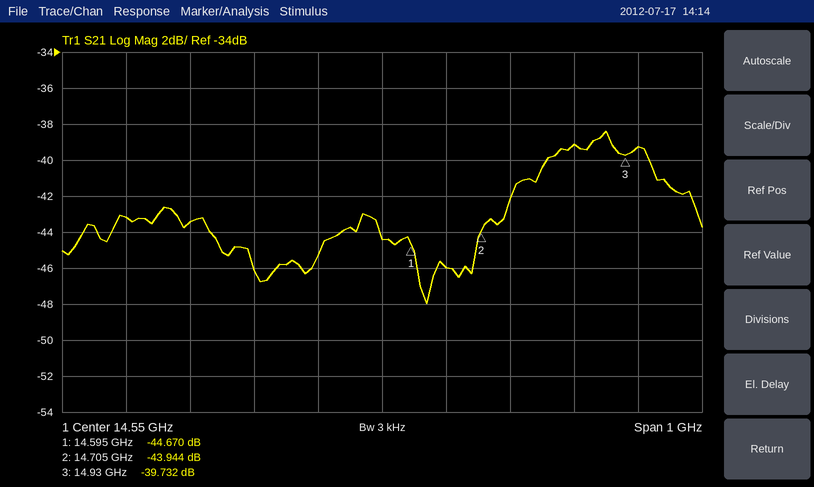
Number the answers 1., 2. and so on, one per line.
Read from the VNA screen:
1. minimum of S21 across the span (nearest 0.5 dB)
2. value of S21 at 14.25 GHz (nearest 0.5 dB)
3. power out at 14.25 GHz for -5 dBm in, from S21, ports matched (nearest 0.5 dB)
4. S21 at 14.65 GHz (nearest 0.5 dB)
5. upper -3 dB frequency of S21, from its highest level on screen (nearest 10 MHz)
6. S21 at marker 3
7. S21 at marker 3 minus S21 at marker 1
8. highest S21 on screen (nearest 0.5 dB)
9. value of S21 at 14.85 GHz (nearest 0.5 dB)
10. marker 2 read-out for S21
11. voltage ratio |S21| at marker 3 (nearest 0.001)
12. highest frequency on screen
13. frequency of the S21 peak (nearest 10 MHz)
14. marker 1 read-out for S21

1. -48.0 dB
2. -43.5 dB
3. -48.5 dBm
4. -46.0 dB
5. 15.00 GHz
6. -39.732 dB
7. 4.938 dB
8. -38.5 dB
9. -39.0 dB
10. -43.944 dB
11. 0.010
12. 15.05 GHz
13. 14.90 GHz
14. -44.670 dB
